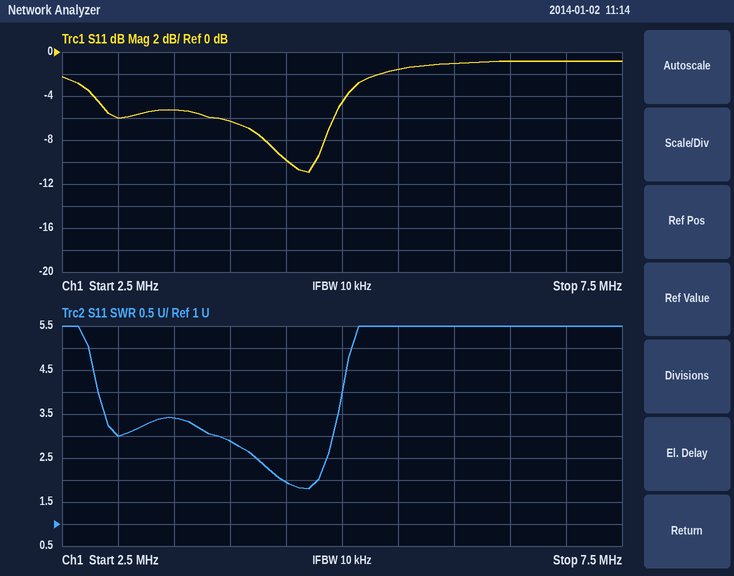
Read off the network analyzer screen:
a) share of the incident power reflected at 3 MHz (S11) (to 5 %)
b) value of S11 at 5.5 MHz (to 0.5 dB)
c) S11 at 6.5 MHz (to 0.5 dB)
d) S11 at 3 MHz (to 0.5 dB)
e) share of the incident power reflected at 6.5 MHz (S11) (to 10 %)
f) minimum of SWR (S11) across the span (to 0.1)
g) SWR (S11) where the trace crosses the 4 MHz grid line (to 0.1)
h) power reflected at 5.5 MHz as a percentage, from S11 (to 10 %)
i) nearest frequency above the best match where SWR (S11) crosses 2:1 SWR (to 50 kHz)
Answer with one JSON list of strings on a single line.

["25 %", "-1.5 dB", "-1.0 dB", "-6.0 dB", "80 %", "1.8", "2.9", "70 %", "4.80 MHz"]
